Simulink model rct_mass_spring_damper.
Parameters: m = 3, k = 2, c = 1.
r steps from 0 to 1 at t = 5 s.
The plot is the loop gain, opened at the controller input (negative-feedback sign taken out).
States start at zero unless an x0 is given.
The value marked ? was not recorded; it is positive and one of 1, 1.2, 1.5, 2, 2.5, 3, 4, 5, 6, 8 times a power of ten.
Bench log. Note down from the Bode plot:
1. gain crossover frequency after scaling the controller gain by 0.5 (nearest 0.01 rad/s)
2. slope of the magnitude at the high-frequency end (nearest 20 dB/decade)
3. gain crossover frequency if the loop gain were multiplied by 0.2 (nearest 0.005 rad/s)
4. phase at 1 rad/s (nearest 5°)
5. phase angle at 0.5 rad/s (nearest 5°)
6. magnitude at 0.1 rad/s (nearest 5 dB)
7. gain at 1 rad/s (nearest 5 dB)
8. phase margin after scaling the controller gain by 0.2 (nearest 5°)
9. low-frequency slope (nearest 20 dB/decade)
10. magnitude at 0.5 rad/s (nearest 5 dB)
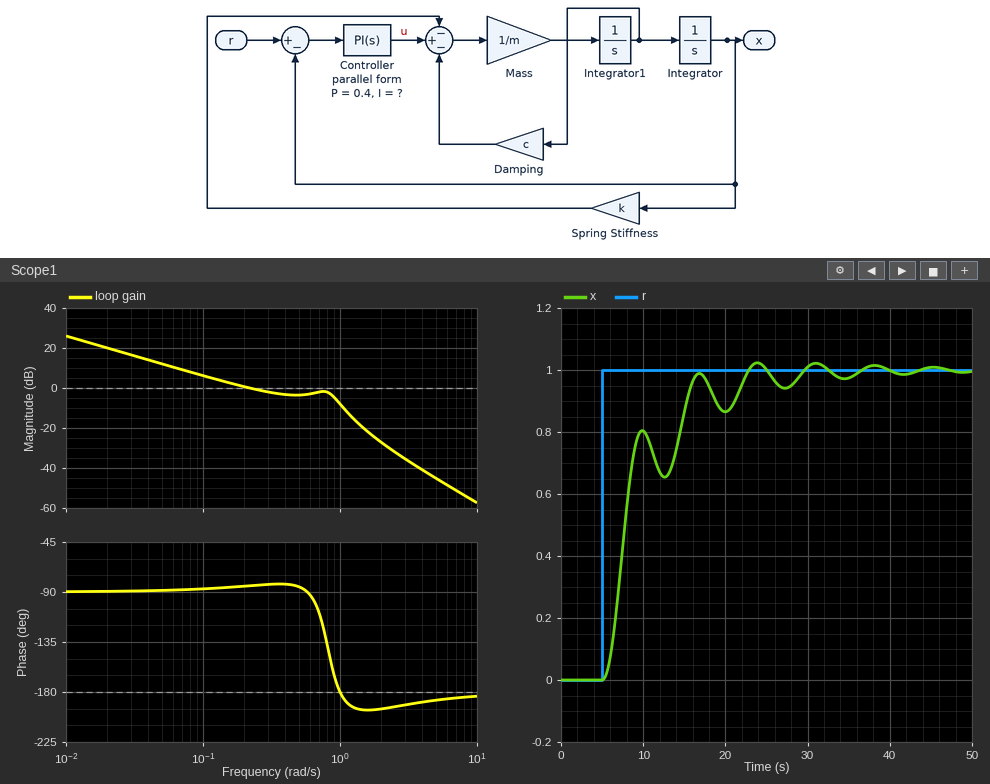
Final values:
0.10 rad/s
-40 dB/decade
0.040 rad/s
-180°
-85°
5 dB
-10 dB
90°
-20 dB/decade
-5 dB
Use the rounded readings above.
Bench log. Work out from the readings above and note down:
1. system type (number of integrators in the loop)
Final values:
1
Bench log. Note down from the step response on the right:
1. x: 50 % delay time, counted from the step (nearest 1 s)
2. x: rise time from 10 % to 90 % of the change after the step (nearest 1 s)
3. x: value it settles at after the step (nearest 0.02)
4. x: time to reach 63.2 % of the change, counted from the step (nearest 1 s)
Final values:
3 s
9 s
1.00
3 s
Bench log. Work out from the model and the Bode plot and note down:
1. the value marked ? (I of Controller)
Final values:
0.4
